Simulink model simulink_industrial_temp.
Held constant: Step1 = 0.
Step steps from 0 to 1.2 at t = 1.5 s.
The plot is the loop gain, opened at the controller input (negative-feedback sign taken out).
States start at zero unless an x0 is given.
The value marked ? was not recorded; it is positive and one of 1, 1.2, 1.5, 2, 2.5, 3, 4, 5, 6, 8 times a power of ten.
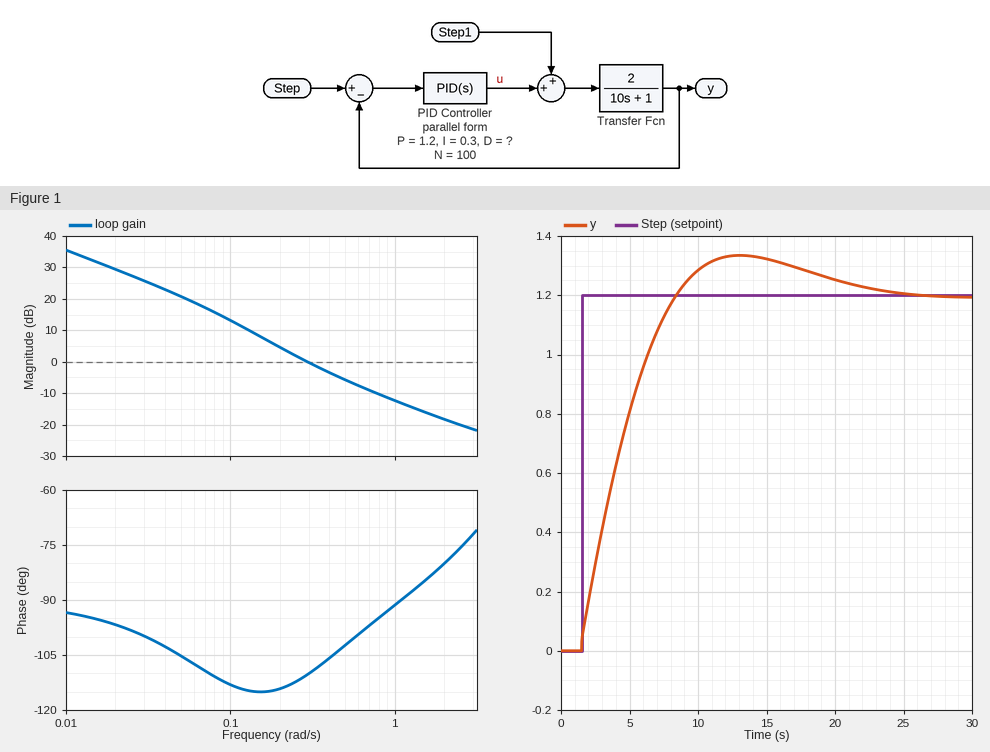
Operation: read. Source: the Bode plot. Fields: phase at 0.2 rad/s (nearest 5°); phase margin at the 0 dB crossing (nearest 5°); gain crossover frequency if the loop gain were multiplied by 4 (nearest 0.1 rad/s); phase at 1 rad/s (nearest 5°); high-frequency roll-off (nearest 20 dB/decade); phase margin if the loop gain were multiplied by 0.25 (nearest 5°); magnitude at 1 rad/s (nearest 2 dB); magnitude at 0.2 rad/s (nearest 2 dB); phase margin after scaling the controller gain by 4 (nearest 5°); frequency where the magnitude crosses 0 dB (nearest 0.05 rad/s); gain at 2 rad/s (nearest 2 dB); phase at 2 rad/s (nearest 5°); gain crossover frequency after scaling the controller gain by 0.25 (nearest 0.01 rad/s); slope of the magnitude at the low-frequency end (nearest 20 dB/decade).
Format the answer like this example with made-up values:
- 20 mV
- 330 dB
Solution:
- -115°
- 70°
- 1.0 rad/s
- -90°
- -20 dB/decade
- 65°
- -12 dB
- 4 dB
- 90°
- 0.30 rad/s
- -18 dB
- -80°
- 0.11 rad/s
- -20 dB/decade
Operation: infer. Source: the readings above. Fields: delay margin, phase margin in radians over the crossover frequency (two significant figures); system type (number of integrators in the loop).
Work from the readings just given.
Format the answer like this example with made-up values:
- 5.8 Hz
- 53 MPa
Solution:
- 4.1 s
- 1
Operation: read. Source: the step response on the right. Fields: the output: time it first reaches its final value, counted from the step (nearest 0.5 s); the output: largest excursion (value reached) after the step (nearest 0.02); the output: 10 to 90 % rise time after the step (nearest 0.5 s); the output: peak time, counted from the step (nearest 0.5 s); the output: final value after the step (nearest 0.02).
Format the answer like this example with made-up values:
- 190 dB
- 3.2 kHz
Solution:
- 7.0 s
- 1.34
- 5.0 s
- 11.5 s
- 1.20
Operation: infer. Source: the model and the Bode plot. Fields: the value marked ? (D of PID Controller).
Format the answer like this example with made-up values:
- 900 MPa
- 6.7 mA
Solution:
- 0.15
